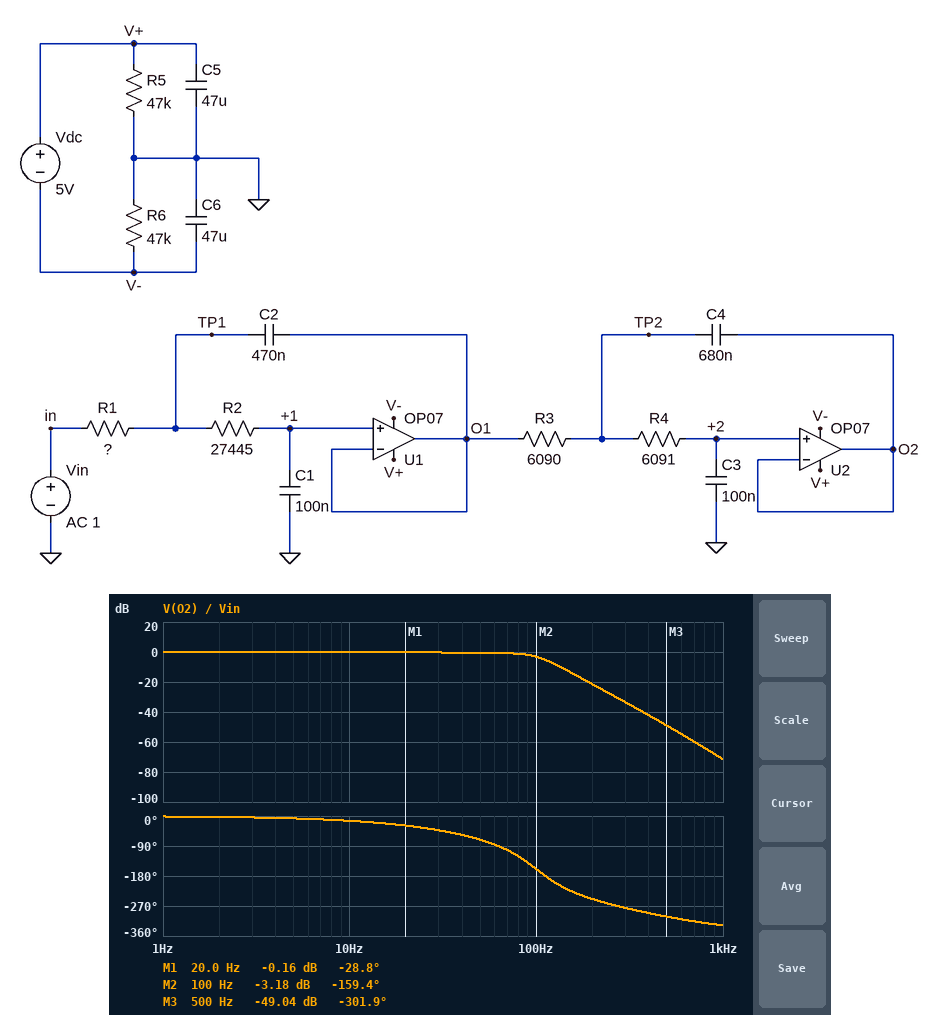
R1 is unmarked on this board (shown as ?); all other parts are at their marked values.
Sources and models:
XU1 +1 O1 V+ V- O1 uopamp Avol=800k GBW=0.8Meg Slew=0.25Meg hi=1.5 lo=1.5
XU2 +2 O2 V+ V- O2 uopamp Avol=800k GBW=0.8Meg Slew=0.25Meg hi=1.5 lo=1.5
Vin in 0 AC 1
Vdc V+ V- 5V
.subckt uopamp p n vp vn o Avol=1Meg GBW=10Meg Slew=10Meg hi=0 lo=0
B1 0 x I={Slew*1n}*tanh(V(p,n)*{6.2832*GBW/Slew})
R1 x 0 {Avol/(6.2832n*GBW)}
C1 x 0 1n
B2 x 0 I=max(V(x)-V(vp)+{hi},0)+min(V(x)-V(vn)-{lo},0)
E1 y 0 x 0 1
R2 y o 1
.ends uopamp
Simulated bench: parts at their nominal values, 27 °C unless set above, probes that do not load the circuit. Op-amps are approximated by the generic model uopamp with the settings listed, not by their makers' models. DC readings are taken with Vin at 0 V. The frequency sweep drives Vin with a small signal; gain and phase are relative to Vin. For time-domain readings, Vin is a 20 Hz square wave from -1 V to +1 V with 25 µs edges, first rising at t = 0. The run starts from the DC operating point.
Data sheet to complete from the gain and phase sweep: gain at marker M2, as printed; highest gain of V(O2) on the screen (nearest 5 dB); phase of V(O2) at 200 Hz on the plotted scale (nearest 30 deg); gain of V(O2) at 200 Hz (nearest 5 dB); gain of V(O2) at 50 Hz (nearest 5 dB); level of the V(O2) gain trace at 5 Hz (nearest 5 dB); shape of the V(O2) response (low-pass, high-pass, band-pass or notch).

-3.18 dB
0 dB
-240 deg
-20 dB
0 dB
0 dB
low-pass
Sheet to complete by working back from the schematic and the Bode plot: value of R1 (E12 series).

680 Ω
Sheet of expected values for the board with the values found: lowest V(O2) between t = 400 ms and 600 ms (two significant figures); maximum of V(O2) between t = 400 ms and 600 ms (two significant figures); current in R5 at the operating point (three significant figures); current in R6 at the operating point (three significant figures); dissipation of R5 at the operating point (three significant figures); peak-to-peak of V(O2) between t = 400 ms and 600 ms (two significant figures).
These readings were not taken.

-1.0 V
1.0 V
53.2 µA
53.2 µA
133 µW
2.0 V
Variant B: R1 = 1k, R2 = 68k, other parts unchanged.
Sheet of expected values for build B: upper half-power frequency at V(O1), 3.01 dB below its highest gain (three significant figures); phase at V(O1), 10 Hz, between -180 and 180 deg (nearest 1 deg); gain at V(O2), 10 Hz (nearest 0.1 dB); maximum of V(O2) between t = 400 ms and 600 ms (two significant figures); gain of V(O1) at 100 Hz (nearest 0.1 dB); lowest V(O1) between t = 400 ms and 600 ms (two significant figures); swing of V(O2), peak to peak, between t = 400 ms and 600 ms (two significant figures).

24.7 Hz
-24 deg
-0.6 dB
950 mV
-12.8 dB
-960 mV
1.9 V
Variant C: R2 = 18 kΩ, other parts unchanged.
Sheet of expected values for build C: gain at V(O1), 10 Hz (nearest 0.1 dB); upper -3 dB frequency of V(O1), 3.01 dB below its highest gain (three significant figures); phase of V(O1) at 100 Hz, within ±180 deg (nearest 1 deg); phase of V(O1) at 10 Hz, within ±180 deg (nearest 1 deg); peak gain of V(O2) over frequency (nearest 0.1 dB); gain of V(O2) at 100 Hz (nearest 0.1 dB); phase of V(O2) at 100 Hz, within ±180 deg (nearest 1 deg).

0 dB
101 Hz
-57 deg
-7 deg
1.0 dB
-0.6 dB
-146 deg
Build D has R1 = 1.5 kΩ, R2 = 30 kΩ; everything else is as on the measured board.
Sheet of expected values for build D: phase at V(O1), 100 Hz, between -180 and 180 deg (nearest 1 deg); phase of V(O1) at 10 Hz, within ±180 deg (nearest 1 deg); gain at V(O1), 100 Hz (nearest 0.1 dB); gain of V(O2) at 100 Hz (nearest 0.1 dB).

-85 deg
-11 deg
-6.0 dB
-3.6 dB
